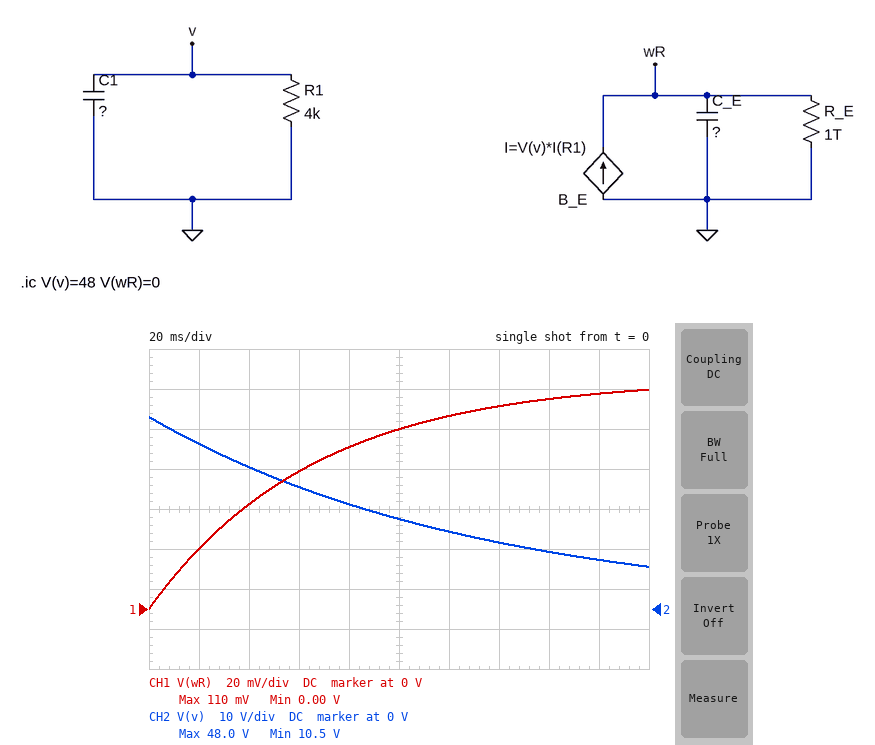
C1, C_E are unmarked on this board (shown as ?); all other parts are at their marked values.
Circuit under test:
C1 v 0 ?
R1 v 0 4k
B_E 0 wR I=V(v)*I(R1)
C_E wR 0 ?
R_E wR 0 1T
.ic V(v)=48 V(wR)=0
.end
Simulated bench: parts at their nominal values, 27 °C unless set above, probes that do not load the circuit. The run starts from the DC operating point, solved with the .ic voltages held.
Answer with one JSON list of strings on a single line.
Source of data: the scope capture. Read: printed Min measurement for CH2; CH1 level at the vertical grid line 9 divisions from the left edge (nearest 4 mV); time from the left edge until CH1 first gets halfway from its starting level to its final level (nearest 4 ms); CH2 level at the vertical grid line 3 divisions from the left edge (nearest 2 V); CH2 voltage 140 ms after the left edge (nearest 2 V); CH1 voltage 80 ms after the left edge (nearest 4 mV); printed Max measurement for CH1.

["10.5 V", "108 mV", "44 ms", "30 V", "16 V", "80 mV", "110 mV"]
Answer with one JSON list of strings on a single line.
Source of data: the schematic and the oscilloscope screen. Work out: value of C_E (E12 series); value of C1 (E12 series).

["330 mF", "33 µF"]
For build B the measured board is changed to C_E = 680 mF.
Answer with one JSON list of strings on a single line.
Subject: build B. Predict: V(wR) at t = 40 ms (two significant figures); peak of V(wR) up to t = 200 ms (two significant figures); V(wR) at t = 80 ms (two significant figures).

["25 mV", "53 mV", "39 mV"]
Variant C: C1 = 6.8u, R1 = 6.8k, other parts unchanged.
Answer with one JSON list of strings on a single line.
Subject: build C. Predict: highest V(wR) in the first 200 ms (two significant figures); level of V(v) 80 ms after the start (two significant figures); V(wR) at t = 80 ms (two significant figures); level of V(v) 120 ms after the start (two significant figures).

["24 mV", "8.5 V", "23 mV", "3.6 V"]
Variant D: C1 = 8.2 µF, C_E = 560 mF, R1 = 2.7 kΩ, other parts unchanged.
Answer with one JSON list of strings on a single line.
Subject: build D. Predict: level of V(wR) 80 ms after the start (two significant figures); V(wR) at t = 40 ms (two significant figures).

["17 mV", "16 mV"]
